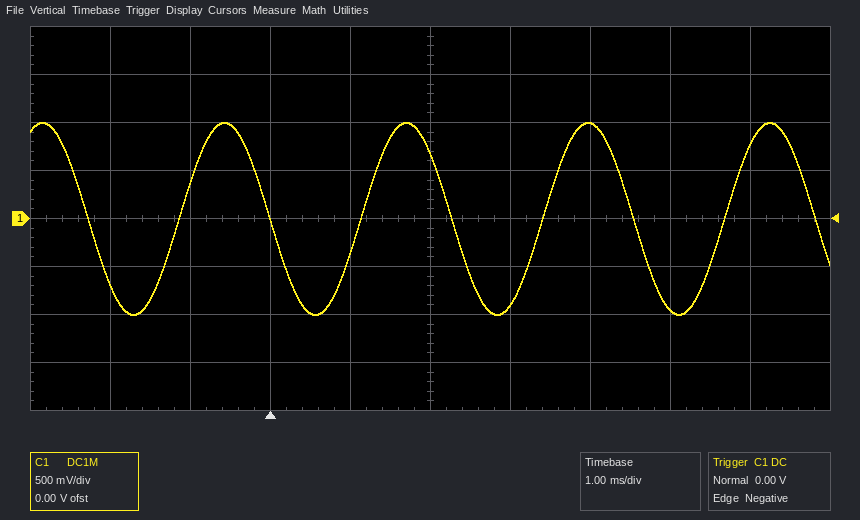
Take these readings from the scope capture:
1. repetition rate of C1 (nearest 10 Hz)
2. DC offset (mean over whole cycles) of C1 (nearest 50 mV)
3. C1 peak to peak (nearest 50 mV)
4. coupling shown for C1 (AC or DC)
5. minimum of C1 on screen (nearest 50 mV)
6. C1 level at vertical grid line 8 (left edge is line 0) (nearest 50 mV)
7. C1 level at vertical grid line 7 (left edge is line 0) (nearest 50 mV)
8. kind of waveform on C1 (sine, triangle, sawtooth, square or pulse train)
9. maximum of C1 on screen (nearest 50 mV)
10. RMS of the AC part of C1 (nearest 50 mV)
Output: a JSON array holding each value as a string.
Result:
["440 Hz", "0 mV", "2.00 V", "DC", "-1.00 V", "-950 mV", "1.00 V", "sine", "1.00 V", "700 mV"]
